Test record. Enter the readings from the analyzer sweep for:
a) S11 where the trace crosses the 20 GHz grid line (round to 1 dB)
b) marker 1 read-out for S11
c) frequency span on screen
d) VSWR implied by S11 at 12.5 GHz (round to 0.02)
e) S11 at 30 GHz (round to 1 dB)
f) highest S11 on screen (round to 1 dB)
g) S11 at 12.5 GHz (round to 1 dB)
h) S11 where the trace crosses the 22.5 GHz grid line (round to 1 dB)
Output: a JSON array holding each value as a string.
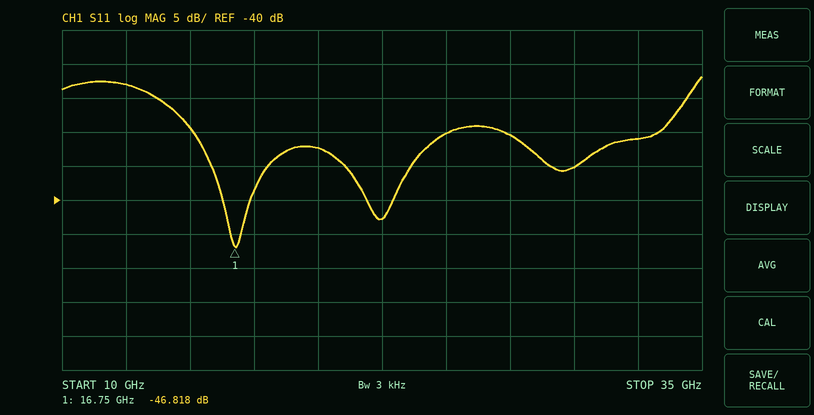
["-32 dB", "-46.818 dB", "25 GHz", "1.16", "-35 dB", "-22 dB", "-23 dB", "-43 dB"]
